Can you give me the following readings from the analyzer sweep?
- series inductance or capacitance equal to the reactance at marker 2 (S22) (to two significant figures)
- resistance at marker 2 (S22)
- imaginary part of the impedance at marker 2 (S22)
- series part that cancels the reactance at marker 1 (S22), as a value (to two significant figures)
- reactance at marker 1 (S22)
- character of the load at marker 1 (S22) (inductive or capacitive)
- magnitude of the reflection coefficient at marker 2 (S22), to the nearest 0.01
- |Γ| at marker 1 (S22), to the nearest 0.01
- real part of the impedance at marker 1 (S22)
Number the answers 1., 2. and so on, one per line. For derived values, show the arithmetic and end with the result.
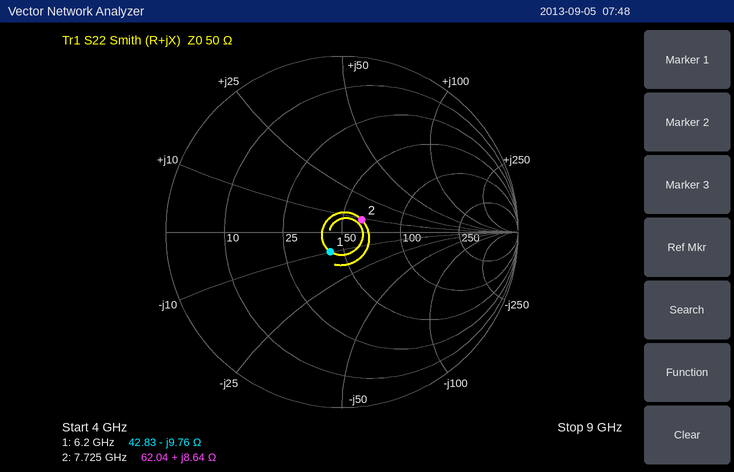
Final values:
1. L = 8.64 Ω/(2π × 7.725 GHz) ≈ 178 pH, so 180 pH to two significant figures
2. 62.04 Ω
3. +8.64 Ω
4. L = 9.76 Ω/(2π × 6.2 GHz) ≈ 251 pH, so 250 pH to two significant figures
5. -9.76 Ω
6. capacitive
7. 0.13
8. 0.13
9. 42.83 Ω
